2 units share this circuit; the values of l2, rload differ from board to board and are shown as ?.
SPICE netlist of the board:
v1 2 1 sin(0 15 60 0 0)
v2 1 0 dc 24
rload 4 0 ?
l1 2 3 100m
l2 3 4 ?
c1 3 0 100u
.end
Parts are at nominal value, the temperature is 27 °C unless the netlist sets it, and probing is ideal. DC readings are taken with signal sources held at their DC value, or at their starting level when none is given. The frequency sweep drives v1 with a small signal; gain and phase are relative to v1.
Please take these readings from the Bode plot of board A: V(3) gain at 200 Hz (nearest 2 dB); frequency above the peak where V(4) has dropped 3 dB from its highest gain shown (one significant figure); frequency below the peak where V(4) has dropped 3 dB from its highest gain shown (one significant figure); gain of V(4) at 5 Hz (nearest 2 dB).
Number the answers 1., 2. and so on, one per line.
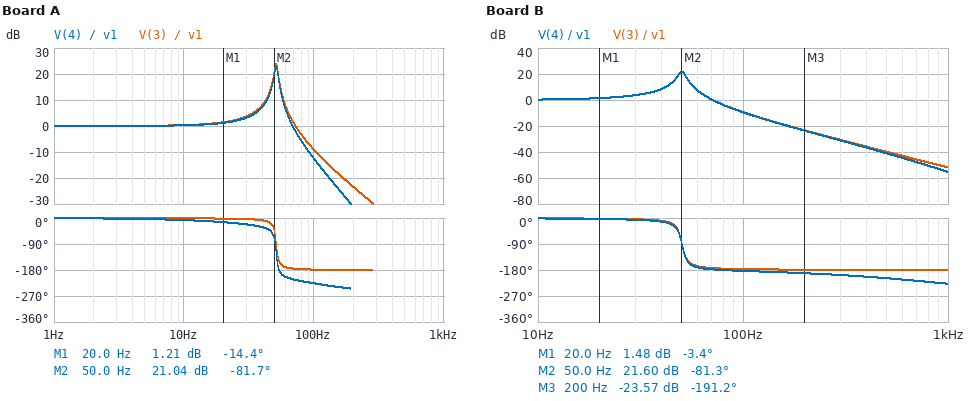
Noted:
1. -24 dB
2. 50 Hz
3. 50 Hz
4. 0 dB
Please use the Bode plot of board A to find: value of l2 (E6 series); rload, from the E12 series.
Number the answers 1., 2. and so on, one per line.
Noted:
1. 680 mH
2. 390 Ω
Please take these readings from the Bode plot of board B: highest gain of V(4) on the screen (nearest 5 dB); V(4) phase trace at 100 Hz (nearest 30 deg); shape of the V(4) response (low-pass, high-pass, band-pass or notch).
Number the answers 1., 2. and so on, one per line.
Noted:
1. 20 dB
2. -180 deg
3. low-pass
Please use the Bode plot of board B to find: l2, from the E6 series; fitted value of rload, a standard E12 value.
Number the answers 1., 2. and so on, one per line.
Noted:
1. 68 mH
2. 390 Ω
